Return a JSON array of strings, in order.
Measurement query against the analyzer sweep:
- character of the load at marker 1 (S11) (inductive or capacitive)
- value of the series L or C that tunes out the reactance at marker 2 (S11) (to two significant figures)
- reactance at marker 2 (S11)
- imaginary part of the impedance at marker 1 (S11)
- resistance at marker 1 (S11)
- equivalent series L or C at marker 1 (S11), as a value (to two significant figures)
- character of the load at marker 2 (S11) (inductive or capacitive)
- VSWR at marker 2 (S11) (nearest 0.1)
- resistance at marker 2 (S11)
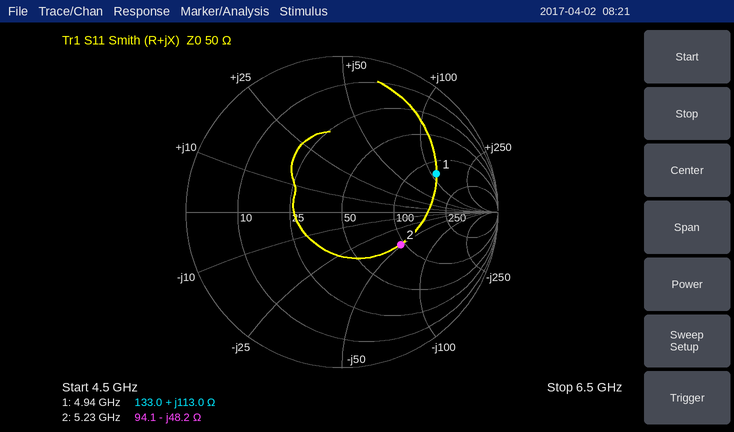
["inductive", "1.5 nH", "-48.2 Ω", "+113.0 Ω", "133.0 Ω", "3.6 nH", "capacitive", "2.5", "94.1 Ω"]
